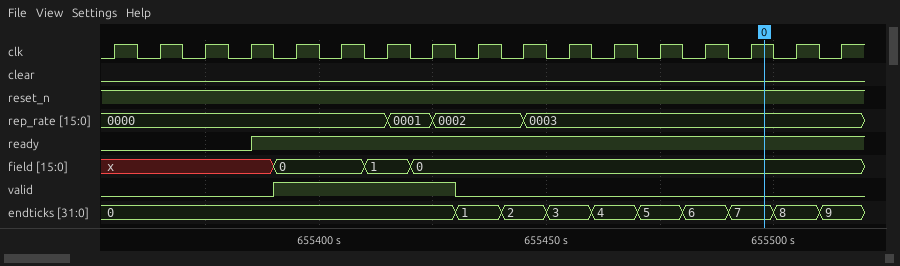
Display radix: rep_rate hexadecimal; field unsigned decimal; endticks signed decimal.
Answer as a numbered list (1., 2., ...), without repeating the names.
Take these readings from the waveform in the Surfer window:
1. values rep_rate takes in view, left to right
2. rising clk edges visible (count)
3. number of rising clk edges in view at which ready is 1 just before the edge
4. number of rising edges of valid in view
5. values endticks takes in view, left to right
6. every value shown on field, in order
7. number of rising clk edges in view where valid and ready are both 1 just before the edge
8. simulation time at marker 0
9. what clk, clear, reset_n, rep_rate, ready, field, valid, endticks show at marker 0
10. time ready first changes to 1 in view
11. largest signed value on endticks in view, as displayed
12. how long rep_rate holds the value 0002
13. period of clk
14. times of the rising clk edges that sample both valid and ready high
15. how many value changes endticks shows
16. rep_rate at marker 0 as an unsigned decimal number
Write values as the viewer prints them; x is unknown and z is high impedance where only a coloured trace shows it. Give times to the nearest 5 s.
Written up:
1. 0000, 0001, 0002, 0003
2. 17
3. 13
4. 1
5. 0, 1, 2, 3, 4, 5, 6, 7, 8, 9
6. x, 0, 1, 0
7. 4
8. 655500 s
9. clk=1, clear=0, reset_n=1, rep_rate=0003, ready=1, field=0, valid=0, endticks=7
10. 655385 s
11. 9
12. 20 s
13. 10 s
14. 655395 s, 655405 s, 655415 s, 655425 s
15. 9
16. 3
